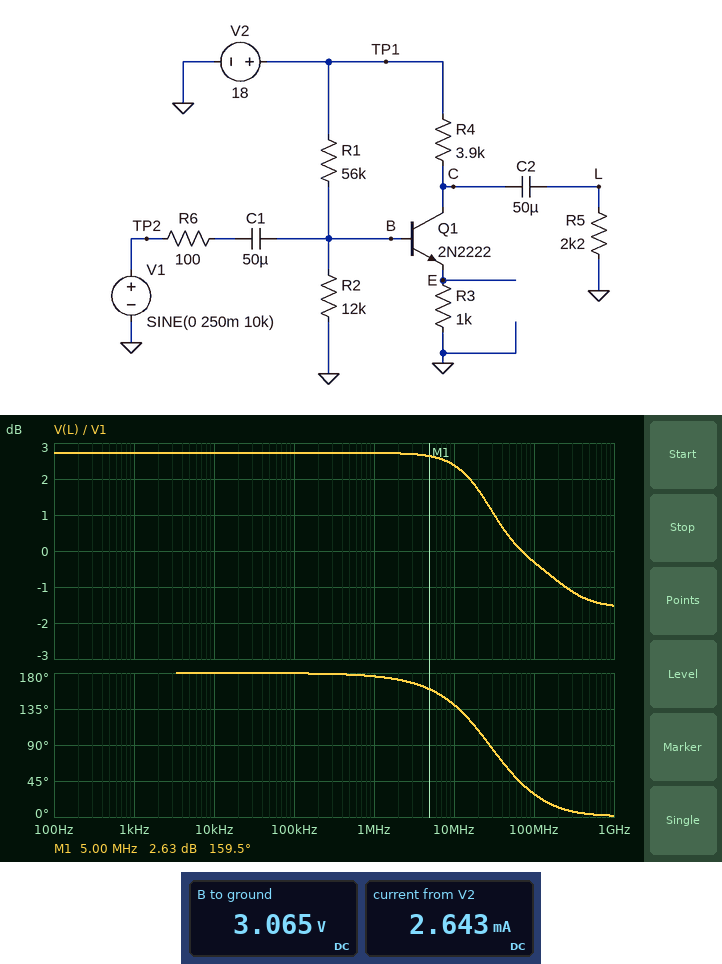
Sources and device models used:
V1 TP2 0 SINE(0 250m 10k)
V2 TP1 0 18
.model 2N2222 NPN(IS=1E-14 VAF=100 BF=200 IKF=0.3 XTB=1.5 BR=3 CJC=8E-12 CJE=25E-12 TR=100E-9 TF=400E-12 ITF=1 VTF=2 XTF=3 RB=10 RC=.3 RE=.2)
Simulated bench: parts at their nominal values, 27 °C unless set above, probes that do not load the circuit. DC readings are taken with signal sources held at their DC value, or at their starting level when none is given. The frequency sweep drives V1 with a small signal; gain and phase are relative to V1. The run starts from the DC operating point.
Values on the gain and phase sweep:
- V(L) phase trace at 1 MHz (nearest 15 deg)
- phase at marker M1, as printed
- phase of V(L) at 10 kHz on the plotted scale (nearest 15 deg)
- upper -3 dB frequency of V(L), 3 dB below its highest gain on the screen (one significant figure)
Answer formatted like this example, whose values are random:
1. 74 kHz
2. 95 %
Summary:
1. 180 deg
2. 159.5 deg
3. 180 deg
4. 100 MHz
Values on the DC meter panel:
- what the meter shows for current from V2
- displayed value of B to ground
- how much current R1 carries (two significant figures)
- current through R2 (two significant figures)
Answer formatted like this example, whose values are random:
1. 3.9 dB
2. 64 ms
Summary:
1. 2.643 mA
2. 3.065 V
3. 270 µA
4. 260 µA
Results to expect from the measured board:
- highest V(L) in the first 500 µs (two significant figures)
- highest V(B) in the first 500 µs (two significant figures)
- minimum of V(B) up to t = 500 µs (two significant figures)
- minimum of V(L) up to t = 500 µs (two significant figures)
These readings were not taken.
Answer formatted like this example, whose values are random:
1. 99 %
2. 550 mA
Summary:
1. 340 mV
2. 3.3 V
3. 2.8 V
4. -340 mV
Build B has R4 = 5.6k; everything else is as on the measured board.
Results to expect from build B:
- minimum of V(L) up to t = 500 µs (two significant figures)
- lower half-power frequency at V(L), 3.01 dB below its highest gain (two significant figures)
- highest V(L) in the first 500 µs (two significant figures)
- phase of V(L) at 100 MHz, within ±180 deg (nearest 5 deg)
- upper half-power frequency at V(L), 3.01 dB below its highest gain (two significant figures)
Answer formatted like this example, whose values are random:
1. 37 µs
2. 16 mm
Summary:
1. -380 mV
2. 580 mHz
3. 380 mV
4. 20 deg
5. 31 MHz
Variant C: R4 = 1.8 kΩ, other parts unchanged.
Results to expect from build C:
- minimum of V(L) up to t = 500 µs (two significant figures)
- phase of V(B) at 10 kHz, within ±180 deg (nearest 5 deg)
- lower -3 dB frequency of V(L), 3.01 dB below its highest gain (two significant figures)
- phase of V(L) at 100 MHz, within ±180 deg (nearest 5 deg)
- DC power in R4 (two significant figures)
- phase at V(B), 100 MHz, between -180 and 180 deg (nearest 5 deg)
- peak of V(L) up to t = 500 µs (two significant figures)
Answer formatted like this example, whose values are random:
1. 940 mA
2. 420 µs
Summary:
1. -240 mV
2. 0 deg
3. 910 mHz
4. 40 deg
5. 10 mW
6. -5 deg
7. 240 mV
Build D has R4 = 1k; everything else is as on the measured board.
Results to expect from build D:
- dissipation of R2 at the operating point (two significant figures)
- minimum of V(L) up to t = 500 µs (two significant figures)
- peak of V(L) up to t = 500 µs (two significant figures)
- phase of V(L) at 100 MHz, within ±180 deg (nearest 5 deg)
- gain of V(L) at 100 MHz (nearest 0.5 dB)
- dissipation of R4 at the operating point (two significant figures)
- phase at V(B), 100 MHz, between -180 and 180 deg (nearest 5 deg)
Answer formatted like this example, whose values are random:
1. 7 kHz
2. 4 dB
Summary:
1. 790 µW
2. -170 mV
3. 170 mV
4. 50 deg
5. -1.5 dB
6. 5.7 mW
7. -5 deg
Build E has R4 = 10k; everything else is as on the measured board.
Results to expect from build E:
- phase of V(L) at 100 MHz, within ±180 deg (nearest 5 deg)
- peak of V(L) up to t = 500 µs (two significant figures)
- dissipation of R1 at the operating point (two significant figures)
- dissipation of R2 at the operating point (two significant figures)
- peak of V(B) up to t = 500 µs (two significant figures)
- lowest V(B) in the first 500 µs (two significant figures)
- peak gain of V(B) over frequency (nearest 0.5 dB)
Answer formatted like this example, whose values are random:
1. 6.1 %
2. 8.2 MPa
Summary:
1. 0 deg
2. 290 mV
3. 4.4 mW
4. 470 µW
5. 2.6 V
6. 2.1 V
7. -1.0 dB
